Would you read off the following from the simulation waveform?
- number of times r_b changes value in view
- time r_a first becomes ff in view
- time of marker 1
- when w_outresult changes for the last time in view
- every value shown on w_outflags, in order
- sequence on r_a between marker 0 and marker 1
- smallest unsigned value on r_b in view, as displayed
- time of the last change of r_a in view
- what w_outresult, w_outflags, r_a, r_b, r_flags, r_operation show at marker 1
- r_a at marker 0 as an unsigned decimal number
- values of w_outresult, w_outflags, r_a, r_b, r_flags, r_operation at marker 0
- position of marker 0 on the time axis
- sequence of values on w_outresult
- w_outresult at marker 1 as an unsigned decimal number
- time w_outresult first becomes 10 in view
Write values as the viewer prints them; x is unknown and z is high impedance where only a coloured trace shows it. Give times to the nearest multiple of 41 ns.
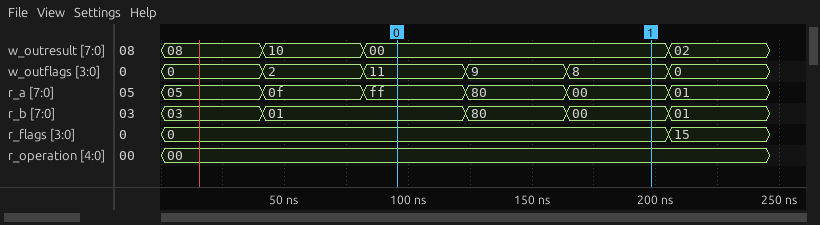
4
82 ns
205 ns
205 ns
0, 2, 11, 9, 8, 0
ff, 80, 00
00
205 ns
w_outresult=00, w_outflags=8, r_a=00, r_b=00, r_flags=0, r_operation=00
255
w_outresult=00, w_outflags=11, r_a=ff, r_b=01, r_flags=0, r_operation=00
82 ns
08, 10, 00, 02
0
41 ns
